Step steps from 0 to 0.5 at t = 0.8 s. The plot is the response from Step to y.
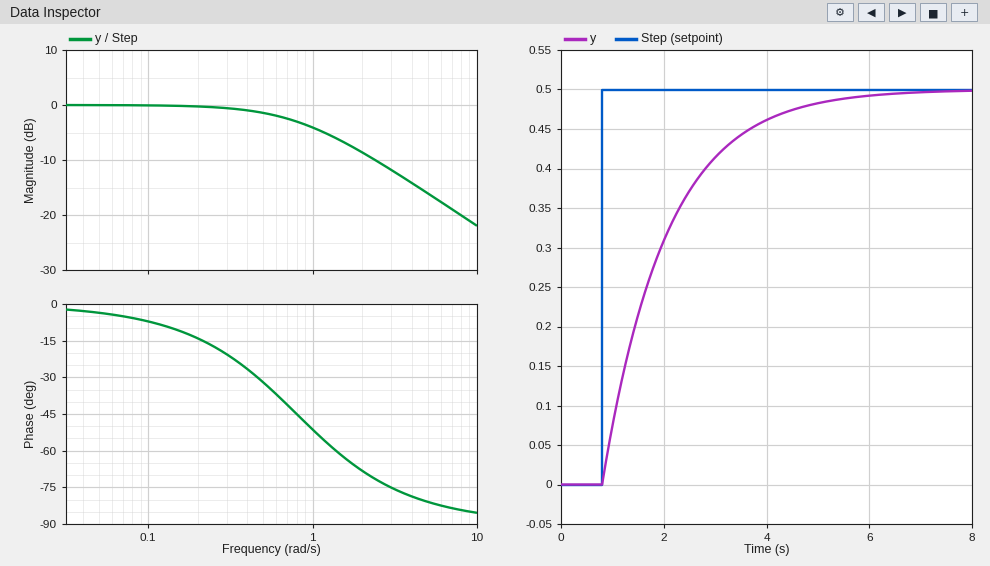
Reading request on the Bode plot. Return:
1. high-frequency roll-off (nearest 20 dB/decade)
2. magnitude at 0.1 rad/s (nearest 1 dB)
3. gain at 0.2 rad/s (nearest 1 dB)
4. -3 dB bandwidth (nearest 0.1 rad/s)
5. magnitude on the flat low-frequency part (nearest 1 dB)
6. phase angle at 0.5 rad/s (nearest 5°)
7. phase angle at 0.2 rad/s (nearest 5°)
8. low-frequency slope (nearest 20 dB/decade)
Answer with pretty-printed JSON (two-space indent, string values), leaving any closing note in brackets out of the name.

{
  "high-frequency roll-off": "-20 dB/decade",
  "magnitude at 0.1 rad/s": "0 dB",
  "gain at 0.2 rad/s": "0 dB",
  "-3 dB bandwidth": "0.8 rad/s",
  "magnitude on the flat low-frequency part": "0 dB",
  "phase angle at 0.5 rad/s": "-30°",
  "phase angle at 0.2 rad/s": "-15°",
  "low-frequency slope": "0 dB/decade"
}
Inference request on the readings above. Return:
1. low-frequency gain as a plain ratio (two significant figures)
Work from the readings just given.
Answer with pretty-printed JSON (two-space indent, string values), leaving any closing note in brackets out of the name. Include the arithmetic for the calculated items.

{
  "low-frequency gain as a plain ratio": "10^(0 / 20) = 1.0"
}
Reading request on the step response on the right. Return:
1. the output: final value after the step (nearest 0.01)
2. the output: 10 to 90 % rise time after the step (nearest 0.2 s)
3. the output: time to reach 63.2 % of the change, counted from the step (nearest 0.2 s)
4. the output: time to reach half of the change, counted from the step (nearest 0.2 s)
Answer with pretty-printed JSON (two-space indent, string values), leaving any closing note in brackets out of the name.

{
  "the output: final value after the step": "0.50",
  "the output: 10 to 90 % rise time after the step": "2.8 s",
  "the output: time to reach 63.2 % of the change, counted from the step": "1.2 s",
  "the output: time to reach half of the change, counted from the step": "0.8 s"
}
